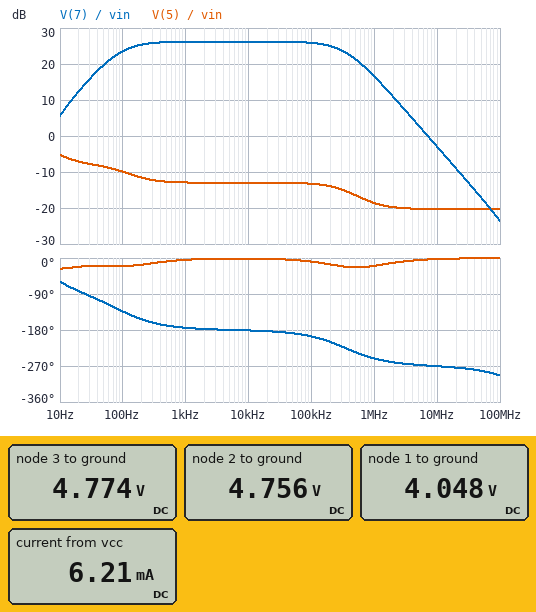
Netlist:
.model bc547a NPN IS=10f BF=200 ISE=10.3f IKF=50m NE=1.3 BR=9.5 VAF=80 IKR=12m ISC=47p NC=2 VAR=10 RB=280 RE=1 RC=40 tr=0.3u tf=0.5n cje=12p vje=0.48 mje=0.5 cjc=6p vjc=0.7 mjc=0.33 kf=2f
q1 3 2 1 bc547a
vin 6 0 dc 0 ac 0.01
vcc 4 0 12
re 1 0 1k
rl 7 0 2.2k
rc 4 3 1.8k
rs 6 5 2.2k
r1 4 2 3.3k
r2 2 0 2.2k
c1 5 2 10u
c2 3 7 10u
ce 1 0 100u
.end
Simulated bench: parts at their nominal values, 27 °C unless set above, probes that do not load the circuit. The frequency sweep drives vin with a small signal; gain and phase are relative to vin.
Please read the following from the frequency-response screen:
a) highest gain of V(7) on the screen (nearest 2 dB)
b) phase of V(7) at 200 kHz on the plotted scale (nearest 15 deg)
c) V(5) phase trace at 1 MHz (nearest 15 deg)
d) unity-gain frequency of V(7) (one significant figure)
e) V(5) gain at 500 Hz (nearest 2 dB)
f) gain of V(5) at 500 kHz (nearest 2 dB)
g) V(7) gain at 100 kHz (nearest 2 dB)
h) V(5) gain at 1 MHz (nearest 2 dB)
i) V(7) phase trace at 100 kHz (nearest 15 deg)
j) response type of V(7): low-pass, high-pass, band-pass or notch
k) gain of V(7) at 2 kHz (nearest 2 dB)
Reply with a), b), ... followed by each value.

a) 26 dB
b) -210 deg
c) -15 deg
d) 7 MHz
e) -12 dB
f) -16 dB
g) 26 dB
h) -18 dB
i) -195 deg
j) band-pass
k) 26 dB
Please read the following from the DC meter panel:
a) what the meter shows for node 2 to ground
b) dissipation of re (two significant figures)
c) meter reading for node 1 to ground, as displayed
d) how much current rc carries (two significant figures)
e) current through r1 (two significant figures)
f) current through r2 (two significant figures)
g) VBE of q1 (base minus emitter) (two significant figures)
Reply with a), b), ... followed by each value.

a) 4.756 V
b) 16 mW
c) 4.048 V
d) 4.0 mA
e) 2.2 mA
f) 2.2 mA
g) 710 mV
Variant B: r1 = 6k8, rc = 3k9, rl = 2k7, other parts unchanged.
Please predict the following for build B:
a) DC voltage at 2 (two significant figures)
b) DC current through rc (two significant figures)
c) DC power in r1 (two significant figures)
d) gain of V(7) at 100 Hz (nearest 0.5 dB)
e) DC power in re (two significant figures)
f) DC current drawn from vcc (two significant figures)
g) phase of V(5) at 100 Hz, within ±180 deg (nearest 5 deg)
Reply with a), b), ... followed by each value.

a) 2.9 V
b) 2.2 mA
c) 12 mW
d) 27.5 dB
e) 4.9 mW
f) 3.5 mA
g) -15 deg
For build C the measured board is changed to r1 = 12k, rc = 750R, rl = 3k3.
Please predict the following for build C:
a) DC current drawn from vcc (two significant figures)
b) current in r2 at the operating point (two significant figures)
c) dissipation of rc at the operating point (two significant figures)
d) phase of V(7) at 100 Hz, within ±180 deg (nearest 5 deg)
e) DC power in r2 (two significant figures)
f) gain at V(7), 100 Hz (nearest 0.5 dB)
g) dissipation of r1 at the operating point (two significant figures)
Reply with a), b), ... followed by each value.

a) 2.0 mA
b) 840 µA
c) 1.0 mW
d) -150 deg
e) 1.5 mW
f) 17.5 dB
g) 8.6 mW
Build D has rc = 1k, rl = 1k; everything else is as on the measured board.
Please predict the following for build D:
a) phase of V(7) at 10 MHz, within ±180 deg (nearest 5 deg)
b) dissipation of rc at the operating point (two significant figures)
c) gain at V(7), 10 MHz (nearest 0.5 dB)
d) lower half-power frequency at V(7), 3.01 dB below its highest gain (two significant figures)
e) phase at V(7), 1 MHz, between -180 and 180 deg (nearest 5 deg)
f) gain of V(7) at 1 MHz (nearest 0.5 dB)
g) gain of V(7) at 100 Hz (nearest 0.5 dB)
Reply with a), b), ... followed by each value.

a) 95 deg
b) 16 mW
c) 0 dB
d) 97 Hz
e) 135 deg
f) 17.5 dB
g) 18.0 dB
